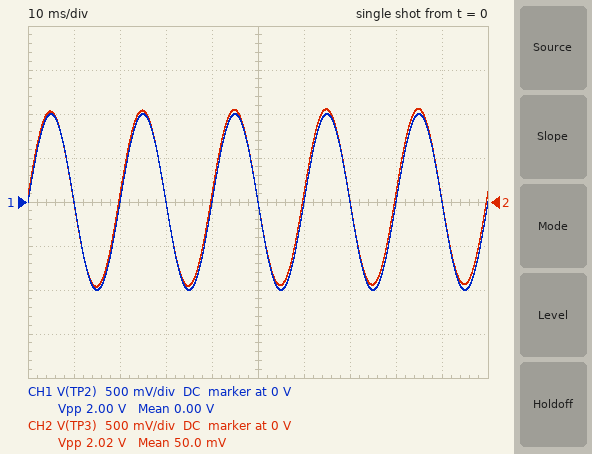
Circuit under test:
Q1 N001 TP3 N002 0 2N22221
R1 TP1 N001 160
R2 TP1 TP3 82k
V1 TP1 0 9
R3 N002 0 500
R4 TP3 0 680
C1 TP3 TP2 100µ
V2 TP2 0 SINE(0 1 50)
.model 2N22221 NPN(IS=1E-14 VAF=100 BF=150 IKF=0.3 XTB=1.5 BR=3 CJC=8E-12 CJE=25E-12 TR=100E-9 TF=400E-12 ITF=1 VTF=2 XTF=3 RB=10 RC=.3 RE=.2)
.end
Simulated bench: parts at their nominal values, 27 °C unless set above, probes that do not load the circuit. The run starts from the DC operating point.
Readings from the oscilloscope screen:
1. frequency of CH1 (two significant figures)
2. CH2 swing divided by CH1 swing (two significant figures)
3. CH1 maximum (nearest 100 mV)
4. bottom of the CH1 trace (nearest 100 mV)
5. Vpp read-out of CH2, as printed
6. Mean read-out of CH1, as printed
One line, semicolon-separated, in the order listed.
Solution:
50 Hz; 1.0; 1.0 V; -1.0 V; 2.02 V; 0.00 V
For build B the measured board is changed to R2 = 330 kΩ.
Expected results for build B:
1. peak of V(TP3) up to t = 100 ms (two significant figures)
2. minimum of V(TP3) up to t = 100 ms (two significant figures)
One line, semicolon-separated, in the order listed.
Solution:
1.0 V; -1.0 V
